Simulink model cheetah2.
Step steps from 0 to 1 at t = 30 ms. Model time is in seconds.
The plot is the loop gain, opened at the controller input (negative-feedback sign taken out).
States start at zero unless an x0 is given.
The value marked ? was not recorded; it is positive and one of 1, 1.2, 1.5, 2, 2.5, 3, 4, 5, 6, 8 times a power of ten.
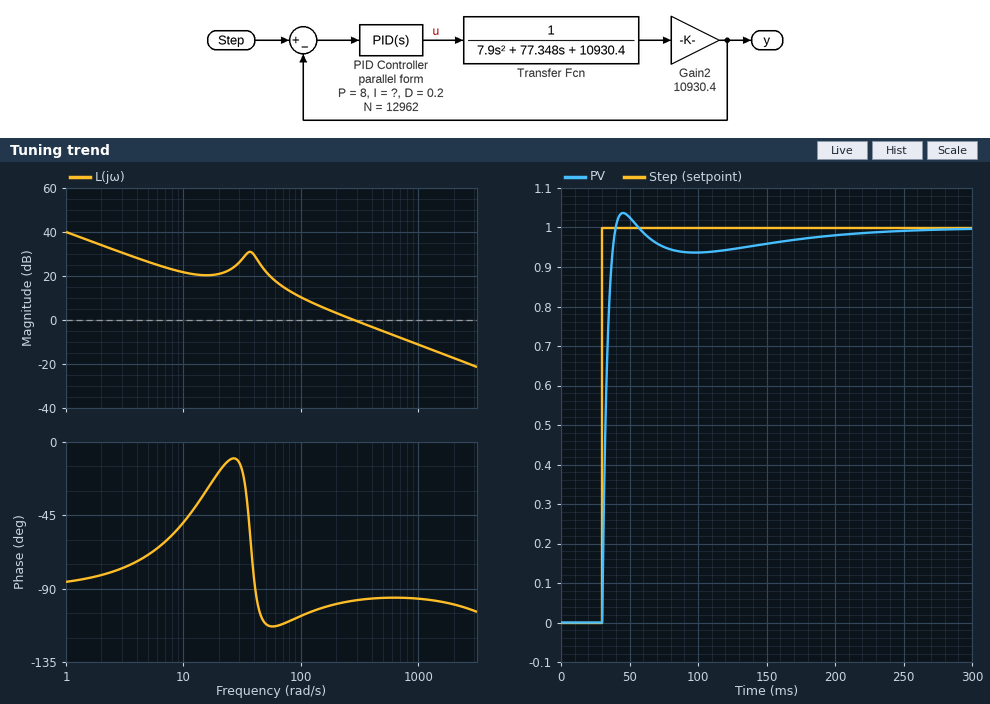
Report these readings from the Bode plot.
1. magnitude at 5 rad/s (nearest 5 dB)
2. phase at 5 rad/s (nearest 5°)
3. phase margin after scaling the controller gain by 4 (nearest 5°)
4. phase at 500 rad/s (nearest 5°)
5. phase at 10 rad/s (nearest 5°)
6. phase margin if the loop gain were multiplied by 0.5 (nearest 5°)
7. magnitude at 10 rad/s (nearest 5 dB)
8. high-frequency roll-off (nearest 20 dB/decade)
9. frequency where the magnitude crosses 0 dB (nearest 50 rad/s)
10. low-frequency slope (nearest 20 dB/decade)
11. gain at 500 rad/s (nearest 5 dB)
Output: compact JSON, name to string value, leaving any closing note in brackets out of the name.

{"magnitude at 5 rad/s": "25 dB", "phase at 5 rad/s": "-70°", "phase margin after scaling the controller gain by 4": "85°", "phase at 500 rad/s": "-95°", "phase at 10 rad/s": "-50°", "phase margin if the loop gain were multiplied by 0.5": "80°", "magnitude at 10 rad/s": "20 dB", "high-frequency roll-off": "-20 dB/decade", "frequency where the magnitude crosses 0 dB": "300 rad/s", "low-frequency slope": "-20 dB/decade", "gain at 500 rad/s": "-5 dB"}
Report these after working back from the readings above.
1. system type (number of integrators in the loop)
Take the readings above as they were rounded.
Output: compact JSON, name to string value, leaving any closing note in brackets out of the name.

{"system type": "1"}
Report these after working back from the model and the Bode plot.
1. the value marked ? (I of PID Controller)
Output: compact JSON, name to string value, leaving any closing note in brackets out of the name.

{"the value marked ?": "100"}
